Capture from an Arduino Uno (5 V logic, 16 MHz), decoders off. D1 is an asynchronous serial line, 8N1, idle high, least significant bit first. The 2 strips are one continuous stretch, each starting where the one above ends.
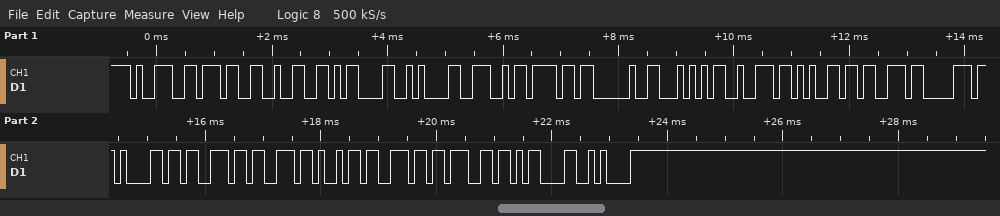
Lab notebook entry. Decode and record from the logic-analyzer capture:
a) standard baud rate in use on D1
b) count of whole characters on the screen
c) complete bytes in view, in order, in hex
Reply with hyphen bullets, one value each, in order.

- 9600 baud
- 21
- 0x39 0x37 0x32 0x0D 0x0A 0x4E 0x6F 0x20 0x54 0x72 0x65 0x73 0x70 0x61 0x73 0x73 0x69 0x6E 0x67 0x0D 0x0A
